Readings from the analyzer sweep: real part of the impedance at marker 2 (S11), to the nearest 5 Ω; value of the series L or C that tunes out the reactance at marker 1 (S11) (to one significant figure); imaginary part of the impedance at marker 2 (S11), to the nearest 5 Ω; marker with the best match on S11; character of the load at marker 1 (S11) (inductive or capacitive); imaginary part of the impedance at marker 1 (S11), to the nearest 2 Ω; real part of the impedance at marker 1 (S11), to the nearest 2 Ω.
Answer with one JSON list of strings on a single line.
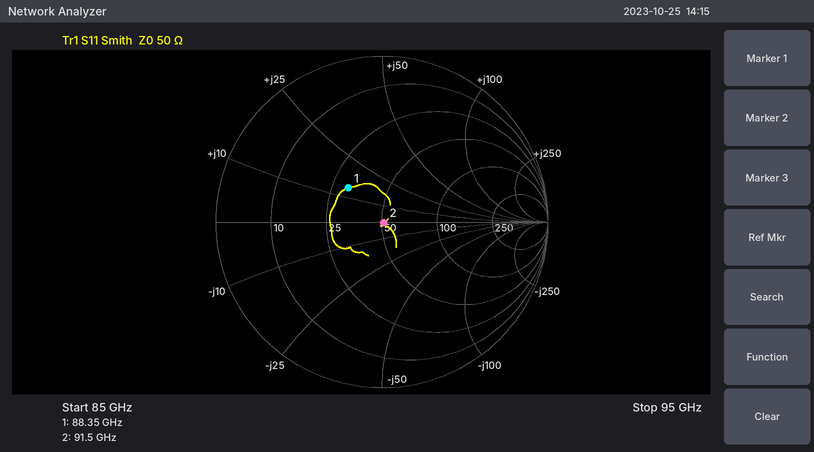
["50 Ω", "100 fF", "0 Ω", "marker 2", "inductive", "+14 Ω", "30 Ω"]
